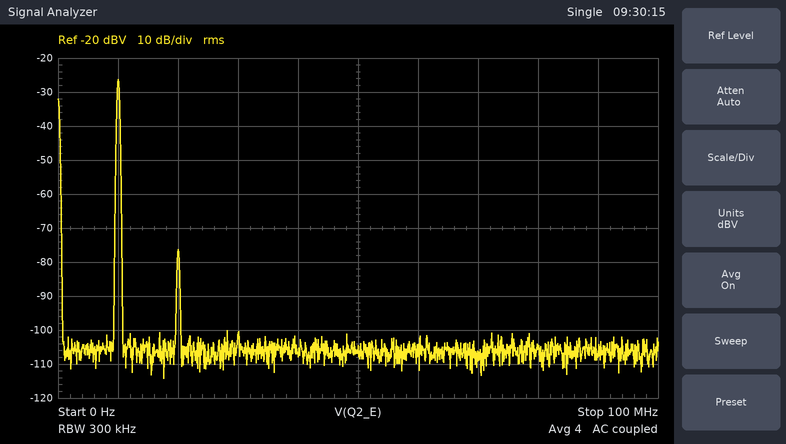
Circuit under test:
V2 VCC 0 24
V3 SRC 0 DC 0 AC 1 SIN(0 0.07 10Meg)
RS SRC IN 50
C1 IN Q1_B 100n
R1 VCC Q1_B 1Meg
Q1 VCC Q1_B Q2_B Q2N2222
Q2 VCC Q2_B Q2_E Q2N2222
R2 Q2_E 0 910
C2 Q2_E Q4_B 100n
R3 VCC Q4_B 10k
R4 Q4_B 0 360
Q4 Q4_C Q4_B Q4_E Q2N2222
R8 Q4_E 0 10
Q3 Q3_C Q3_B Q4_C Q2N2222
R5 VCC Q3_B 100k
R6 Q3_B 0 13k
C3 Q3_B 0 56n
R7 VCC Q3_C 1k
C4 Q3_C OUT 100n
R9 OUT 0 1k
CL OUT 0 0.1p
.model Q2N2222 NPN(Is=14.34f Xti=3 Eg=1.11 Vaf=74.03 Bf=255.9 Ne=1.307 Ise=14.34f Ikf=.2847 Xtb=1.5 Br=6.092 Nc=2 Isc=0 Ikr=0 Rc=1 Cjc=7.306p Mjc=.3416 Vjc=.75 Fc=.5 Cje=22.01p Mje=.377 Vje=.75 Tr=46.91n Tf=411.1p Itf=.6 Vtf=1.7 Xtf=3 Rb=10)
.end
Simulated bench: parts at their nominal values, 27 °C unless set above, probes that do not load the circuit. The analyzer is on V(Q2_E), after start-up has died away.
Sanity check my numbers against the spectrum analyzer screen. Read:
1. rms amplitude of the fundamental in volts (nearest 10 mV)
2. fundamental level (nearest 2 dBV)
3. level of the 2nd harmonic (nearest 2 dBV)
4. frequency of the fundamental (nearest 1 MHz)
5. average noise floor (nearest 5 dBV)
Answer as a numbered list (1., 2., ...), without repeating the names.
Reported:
1. 50 mV
2. -26 dBV
3. -76 dBV
4. 10 MHz
5. -105 dBV
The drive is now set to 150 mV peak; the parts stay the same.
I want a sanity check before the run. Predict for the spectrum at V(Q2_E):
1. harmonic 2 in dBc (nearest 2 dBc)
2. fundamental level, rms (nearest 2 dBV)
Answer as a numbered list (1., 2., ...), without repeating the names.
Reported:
1. -44 dBc
2. -20 dBV
